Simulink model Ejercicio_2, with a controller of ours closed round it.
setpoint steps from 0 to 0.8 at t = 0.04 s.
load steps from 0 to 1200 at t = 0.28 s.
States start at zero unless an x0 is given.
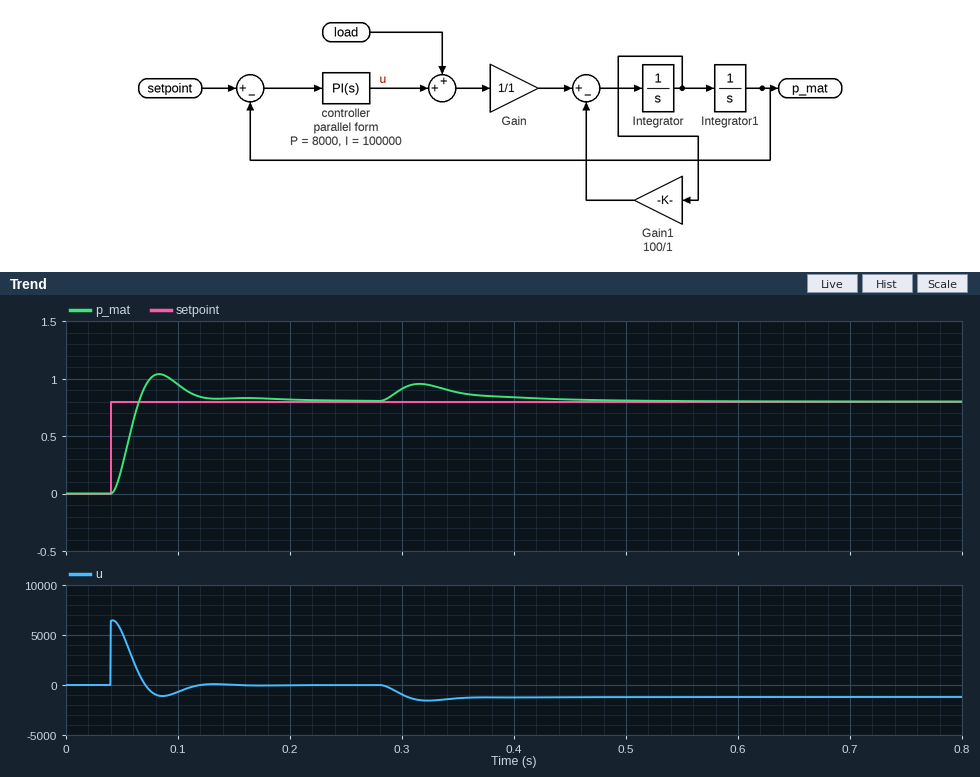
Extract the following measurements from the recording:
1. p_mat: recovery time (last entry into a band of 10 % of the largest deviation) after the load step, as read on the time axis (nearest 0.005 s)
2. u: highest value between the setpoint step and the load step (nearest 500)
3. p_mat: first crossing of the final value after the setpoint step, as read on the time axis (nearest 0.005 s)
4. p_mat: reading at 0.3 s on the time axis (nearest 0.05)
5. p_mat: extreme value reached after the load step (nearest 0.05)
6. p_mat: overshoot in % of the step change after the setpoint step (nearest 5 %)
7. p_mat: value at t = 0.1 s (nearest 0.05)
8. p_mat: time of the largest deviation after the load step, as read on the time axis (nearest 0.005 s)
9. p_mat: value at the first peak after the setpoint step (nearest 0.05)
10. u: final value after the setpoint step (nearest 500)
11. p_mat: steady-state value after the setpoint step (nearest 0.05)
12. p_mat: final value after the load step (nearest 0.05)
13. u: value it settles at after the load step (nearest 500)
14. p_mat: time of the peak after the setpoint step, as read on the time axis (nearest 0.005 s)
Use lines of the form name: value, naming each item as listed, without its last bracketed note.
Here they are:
p_mat: recovery time (last entry into a band of 10 % of the largest deviation) after the load step, as read on the time axis: 0.460 s
u: highest value between the setpoint step and the load step: 6500
p_mat: first crossing of the final value after the setpoint step, as read on the time axis: 0.065 s
p_mat: reading at 0.3 s on the time axis: 0.90
p_mat: extreme value reached after the load step: 0.95
p_mat: overshoot in % of the step change after the setpoint step: 30 %
p_mat: value at t = 0.1 s: 0.95
p_mat: time of the largest deviation after the load step, as read on the time axis: 0.315 s
p_mat: value at the first peak after the setpoint step: 1.05
u: final value after the setpoint step: 0
p_mat: steady-state value after the setpoint step: 0.80
p_mat: final value after the load step: 0.80
u: value it settles at after the load step: -1000
p_mat: time of the peak after the setpoint step, as read on the time axis: 0.085 s
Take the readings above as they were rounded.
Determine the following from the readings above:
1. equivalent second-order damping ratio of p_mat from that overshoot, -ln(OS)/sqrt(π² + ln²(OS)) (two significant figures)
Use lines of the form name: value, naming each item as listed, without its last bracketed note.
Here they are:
equivalent second-order damping ratio of p_mat from that overshoot, -ln(OS)/sqrt(π² + ln²(OS)): 0.36
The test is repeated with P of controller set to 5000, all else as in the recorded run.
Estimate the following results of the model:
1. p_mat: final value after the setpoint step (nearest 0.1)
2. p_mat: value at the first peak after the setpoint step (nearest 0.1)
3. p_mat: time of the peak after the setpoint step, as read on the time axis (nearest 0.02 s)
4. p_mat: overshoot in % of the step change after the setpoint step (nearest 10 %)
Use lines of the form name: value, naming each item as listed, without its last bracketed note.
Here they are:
p_mat: final value after the setpoint step: 0.8
p_mat: value at the first peak after the setpoint step: 1.1
p_mat: time of the peak after the setpoint step, as read on the time axis: 0.10 s
p_mat: overshoot in % of the step change after the setpoint step: 40 %
